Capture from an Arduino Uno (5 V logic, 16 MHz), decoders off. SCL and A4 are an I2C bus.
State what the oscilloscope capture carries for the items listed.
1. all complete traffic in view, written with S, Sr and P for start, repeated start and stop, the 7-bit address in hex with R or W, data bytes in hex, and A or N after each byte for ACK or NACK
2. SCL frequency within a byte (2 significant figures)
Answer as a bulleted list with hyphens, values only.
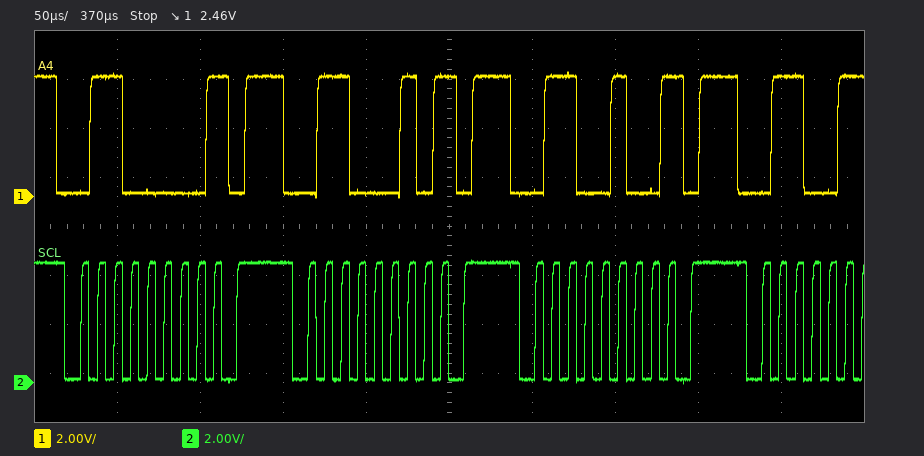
- S 30W N P S 31W N P S 32W N P
- 100 kHz
